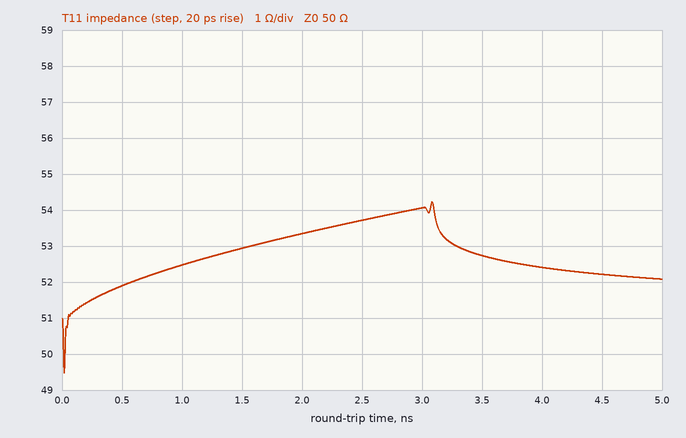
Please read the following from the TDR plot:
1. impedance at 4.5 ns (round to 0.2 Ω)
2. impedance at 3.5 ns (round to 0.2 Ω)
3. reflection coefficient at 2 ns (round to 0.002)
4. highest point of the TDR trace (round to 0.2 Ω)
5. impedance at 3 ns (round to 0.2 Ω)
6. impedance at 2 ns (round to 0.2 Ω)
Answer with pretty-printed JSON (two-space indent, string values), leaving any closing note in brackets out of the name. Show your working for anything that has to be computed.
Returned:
{
  "impedance at 4.5 ns": "52.2 Ω",
  "impedance at 3.5 ns": "52.8 Ω",
  "reflection coefficient at 2 ns": "(53.4 − 50)/(53.4 + 50) ≈ +0.0329, so +0.032 to the nearest 0.002",
  "highest point of the TDR trace": "54.2 Ω",
  "impedance at 3 ns": "54.0 Ω",
  "impedance at 2 ns": "53.4 Ω"
}
